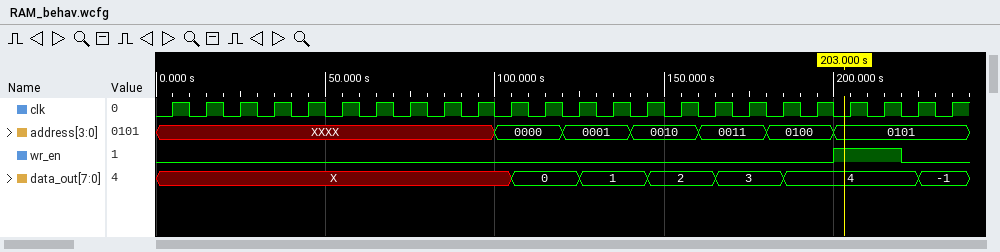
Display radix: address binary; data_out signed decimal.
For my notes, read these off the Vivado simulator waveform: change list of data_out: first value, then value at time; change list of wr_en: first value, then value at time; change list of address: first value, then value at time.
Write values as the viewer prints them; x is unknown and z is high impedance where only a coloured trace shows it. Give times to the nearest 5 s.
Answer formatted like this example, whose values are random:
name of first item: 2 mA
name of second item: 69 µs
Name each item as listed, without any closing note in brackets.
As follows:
change list of data_out: first value, then value at time: X, 0 at 105 s, 1 at 125 s, 2 at 145 s, 3 at 165 s, 4 at 185 s, -1 at 225 s
change list of wr_en: first value, then value at time: 0, 1 at 200 s, 0 at 220 s
change list of address: first value, then value at time: XXXX, 0000 at 100 s, 0001 at 120 s, 0010 at 140 s, 0011 at 160 s, 0100 at 180 s, 0101 at 200 s
